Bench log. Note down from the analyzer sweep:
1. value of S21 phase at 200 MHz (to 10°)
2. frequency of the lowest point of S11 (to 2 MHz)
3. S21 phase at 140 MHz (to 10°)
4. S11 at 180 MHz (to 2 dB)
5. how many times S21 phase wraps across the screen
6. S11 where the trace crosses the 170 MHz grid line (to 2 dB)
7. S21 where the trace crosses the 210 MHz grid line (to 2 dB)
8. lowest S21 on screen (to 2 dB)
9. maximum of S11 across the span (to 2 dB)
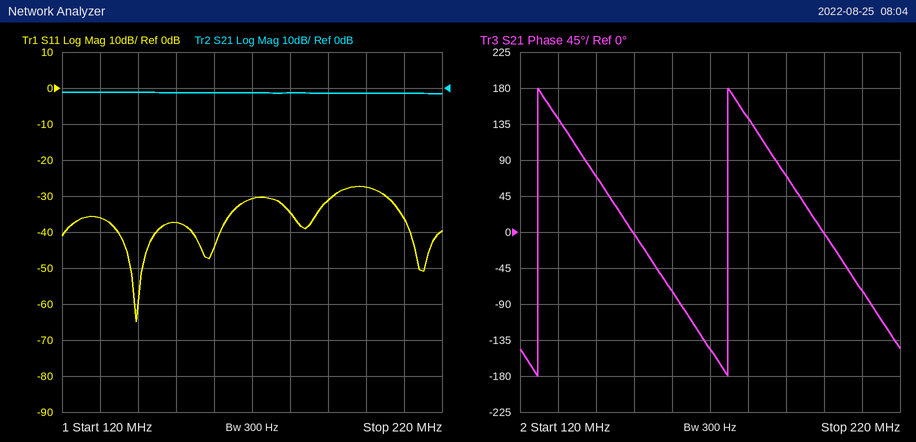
0°
140 MHz
70°
-34 dB
2
-30 dB
-2 dB
-2 dB
-28 dB
